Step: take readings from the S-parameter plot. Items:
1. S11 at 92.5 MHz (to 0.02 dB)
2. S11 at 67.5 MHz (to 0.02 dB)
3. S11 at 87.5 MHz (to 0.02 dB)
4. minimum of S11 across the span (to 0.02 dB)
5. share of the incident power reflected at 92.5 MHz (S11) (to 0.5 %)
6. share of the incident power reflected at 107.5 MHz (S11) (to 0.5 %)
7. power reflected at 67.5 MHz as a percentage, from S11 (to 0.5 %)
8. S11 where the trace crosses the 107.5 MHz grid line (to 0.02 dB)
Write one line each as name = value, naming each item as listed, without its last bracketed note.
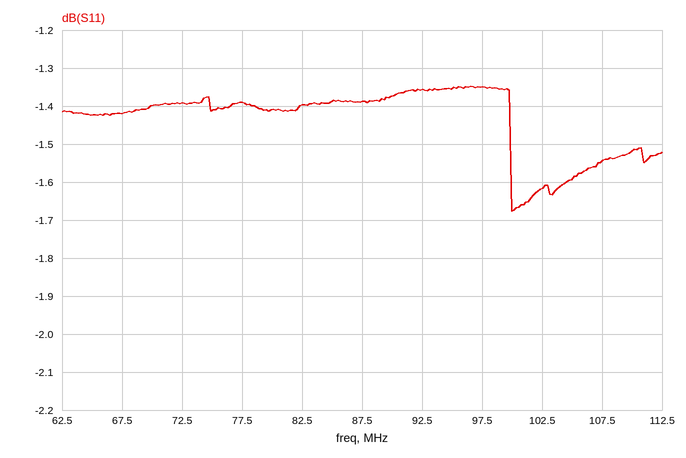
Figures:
S11 at 92.5 MHz = -1.36 dB
S11 at 67.5 MHz = -1.42 dB
S11 at 87.5 MHz = -1.38 dB
minimum of S11 across the span = -1.68 dB
share of the incident power reflected at 92.5 MHz (S11) = 73.0 %
share of the incident power reflected at 107.5 MHz (S11) = 70.0 %
power reflected at 67.5 MHz as a percentage, from S11 = 72.0 %
S11 where the trace crosses the 107.5 MHz grid line = -1.54 dB
